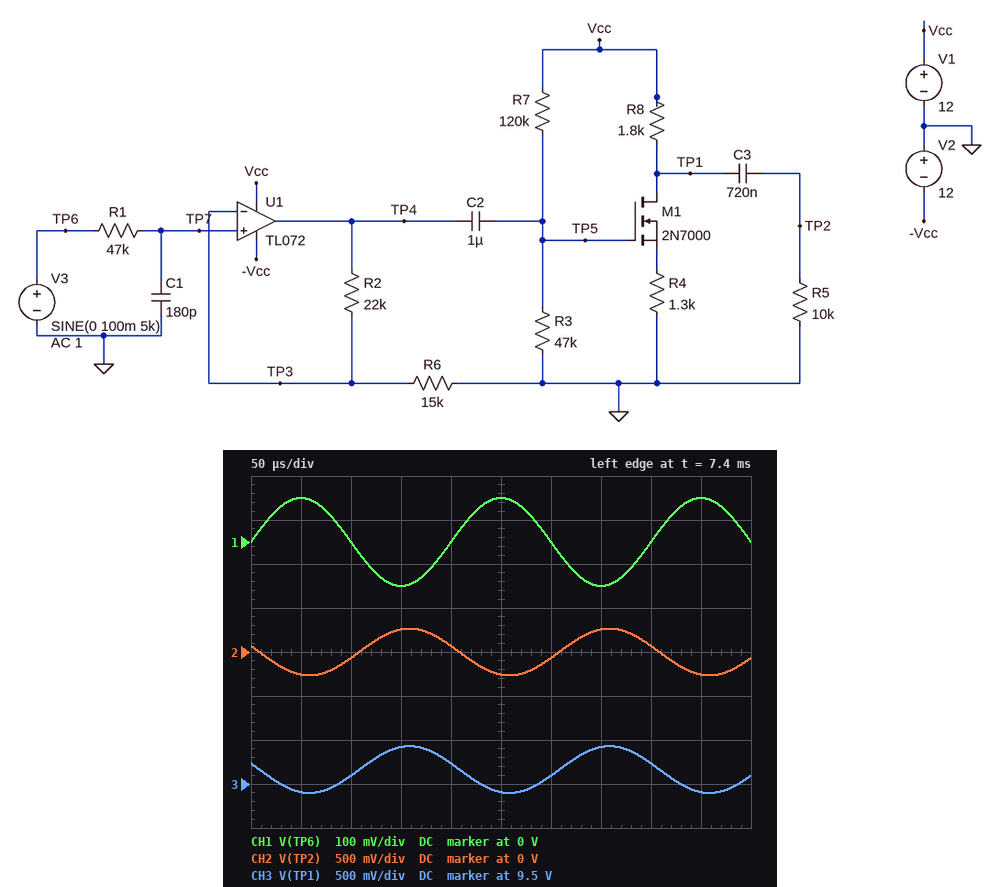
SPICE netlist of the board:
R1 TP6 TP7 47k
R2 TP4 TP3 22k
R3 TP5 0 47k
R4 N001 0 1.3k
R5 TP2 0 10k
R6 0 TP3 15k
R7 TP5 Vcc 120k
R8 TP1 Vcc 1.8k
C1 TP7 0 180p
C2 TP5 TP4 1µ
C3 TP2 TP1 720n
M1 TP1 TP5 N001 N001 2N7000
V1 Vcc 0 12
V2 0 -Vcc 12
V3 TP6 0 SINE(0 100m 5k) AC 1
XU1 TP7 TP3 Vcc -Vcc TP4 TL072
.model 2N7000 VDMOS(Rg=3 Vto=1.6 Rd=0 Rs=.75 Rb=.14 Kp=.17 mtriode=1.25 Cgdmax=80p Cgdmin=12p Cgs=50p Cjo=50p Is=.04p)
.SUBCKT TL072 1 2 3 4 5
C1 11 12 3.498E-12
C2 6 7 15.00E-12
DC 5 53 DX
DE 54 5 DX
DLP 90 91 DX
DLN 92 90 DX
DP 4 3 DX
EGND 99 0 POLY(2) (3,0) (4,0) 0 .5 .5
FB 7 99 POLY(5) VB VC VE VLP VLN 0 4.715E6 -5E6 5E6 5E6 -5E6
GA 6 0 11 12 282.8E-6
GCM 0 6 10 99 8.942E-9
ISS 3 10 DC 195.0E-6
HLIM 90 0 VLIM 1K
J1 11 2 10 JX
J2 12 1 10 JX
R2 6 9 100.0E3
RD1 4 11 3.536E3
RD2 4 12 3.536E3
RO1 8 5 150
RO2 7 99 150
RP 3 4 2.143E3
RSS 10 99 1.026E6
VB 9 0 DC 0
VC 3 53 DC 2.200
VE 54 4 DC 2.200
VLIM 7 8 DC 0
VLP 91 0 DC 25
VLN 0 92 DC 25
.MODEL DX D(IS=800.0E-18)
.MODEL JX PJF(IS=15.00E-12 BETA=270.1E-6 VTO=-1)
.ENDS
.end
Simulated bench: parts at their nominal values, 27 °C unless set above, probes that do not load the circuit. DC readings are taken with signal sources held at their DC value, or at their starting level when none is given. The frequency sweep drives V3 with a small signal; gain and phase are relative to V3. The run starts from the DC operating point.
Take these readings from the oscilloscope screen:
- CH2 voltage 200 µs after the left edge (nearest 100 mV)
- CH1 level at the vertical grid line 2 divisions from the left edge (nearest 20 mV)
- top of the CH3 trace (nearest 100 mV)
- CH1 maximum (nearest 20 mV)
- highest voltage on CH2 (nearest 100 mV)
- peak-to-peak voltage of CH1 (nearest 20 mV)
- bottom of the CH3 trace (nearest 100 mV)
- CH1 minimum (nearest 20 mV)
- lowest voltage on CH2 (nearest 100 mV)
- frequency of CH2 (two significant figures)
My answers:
100 mV
0 V
9.9 V
100 mV
300 mV
200 mV
9.4 V
-100 mV
-300 mV
5.0 kHz
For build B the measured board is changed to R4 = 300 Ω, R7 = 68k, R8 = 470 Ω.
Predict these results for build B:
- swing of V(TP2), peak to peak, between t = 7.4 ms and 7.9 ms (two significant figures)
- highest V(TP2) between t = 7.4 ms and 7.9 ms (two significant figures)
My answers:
670 mV
340 mV
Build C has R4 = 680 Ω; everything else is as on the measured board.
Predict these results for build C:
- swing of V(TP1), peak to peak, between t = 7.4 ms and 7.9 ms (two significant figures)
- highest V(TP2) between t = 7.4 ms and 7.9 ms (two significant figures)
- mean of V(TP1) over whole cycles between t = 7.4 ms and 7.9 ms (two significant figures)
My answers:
1.0 V
500 mV
7.7 V
